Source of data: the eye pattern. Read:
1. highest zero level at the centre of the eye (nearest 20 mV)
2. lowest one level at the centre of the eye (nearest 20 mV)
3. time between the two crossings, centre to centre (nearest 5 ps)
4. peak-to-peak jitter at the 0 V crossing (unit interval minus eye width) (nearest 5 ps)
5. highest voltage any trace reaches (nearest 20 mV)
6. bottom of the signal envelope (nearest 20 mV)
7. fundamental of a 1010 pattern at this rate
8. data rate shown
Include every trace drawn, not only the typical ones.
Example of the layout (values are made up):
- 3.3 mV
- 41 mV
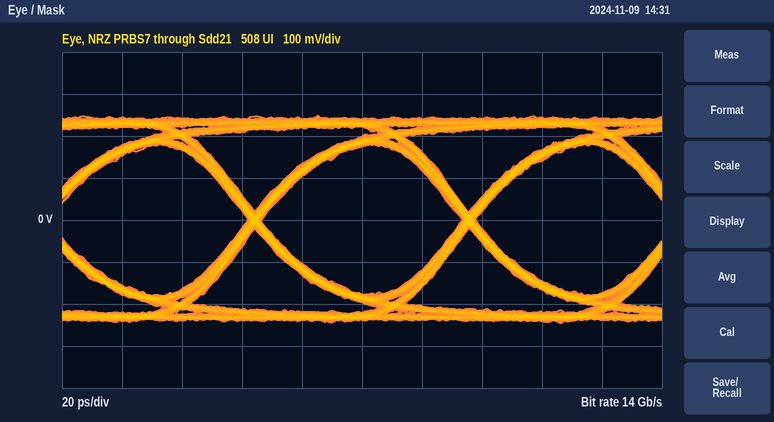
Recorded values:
- -180 mV
- 180 mV
- 70 ps
- 5 ps
- 240 mV
- -240 mV
- 7 GHz
- 14 Gb/s
